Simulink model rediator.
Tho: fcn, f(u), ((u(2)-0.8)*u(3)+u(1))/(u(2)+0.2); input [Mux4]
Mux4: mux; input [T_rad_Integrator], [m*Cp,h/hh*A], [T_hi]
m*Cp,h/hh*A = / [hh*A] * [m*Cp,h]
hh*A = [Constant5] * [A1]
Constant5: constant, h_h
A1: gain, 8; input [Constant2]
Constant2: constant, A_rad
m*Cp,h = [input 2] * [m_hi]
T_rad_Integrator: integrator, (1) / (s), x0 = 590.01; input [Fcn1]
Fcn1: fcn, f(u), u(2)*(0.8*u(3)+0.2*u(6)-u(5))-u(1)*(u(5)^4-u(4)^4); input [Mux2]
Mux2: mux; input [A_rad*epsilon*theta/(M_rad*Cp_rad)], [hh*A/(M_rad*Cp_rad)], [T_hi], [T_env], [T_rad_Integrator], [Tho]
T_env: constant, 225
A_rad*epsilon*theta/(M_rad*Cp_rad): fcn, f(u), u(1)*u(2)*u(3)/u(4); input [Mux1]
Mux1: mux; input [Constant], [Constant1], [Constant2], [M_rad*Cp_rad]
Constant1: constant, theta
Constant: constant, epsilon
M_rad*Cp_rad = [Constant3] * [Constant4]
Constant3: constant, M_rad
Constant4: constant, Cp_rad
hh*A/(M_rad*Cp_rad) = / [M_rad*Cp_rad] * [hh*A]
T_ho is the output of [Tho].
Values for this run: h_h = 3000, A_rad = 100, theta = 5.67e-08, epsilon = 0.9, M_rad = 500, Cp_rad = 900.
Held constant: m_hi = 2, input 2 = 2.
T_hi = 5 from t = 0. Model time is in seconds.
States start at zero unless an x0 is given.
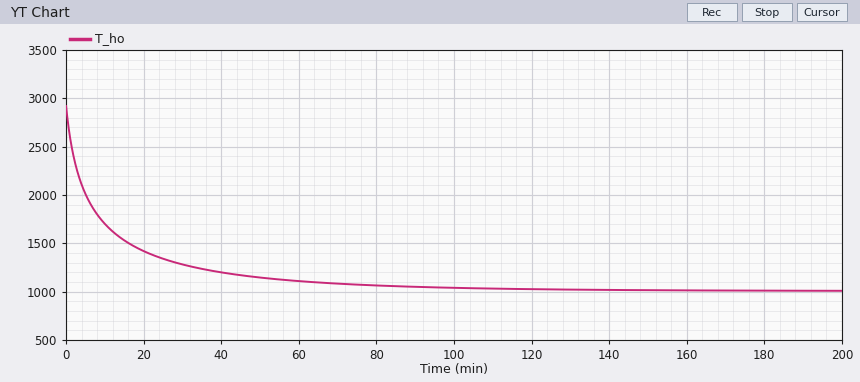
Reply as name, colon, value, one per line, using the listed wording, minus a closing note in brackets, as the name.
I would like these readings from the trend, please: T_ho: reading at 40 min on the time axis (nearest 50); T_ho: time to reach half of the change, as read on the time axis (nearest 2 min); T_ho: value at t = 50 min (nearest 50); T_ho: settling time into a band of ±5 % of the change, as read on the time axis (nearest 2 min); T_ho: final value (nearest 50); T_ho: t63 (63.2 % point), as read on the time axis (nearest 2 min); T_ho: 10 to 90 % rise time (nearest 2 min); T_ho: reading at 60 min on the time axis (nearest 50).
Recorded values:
T_ho: reading at 40 min on the time axis: 1200
T_ho: time to reach half of the change, as read on the time axis: 6 min
T_ho: value at t = 50 min: 1150
T_ho: settling time into a band of ±5 % of the change, as read on the time axis: 62 min
T_ho: final value: 1000
T_ho: t63 (63.2 % point), as read on the time axis: 10 min
T_ho: 10 to 90 % rise time: 40 min
T_ho: reading at 60 min on the time axis: 1100
